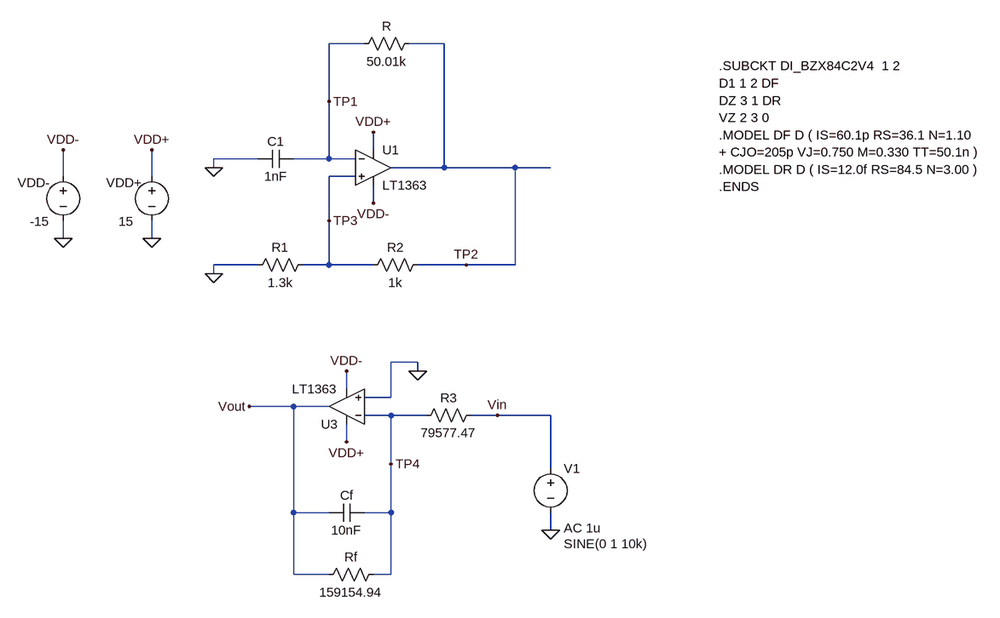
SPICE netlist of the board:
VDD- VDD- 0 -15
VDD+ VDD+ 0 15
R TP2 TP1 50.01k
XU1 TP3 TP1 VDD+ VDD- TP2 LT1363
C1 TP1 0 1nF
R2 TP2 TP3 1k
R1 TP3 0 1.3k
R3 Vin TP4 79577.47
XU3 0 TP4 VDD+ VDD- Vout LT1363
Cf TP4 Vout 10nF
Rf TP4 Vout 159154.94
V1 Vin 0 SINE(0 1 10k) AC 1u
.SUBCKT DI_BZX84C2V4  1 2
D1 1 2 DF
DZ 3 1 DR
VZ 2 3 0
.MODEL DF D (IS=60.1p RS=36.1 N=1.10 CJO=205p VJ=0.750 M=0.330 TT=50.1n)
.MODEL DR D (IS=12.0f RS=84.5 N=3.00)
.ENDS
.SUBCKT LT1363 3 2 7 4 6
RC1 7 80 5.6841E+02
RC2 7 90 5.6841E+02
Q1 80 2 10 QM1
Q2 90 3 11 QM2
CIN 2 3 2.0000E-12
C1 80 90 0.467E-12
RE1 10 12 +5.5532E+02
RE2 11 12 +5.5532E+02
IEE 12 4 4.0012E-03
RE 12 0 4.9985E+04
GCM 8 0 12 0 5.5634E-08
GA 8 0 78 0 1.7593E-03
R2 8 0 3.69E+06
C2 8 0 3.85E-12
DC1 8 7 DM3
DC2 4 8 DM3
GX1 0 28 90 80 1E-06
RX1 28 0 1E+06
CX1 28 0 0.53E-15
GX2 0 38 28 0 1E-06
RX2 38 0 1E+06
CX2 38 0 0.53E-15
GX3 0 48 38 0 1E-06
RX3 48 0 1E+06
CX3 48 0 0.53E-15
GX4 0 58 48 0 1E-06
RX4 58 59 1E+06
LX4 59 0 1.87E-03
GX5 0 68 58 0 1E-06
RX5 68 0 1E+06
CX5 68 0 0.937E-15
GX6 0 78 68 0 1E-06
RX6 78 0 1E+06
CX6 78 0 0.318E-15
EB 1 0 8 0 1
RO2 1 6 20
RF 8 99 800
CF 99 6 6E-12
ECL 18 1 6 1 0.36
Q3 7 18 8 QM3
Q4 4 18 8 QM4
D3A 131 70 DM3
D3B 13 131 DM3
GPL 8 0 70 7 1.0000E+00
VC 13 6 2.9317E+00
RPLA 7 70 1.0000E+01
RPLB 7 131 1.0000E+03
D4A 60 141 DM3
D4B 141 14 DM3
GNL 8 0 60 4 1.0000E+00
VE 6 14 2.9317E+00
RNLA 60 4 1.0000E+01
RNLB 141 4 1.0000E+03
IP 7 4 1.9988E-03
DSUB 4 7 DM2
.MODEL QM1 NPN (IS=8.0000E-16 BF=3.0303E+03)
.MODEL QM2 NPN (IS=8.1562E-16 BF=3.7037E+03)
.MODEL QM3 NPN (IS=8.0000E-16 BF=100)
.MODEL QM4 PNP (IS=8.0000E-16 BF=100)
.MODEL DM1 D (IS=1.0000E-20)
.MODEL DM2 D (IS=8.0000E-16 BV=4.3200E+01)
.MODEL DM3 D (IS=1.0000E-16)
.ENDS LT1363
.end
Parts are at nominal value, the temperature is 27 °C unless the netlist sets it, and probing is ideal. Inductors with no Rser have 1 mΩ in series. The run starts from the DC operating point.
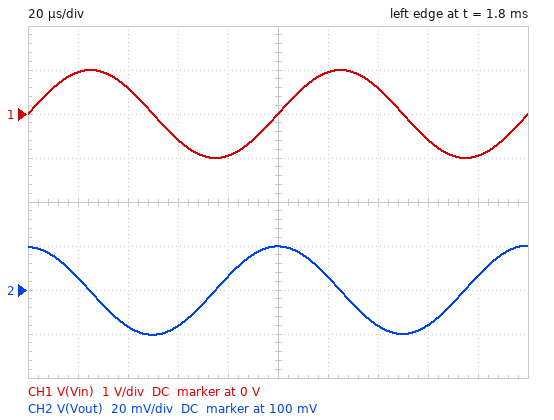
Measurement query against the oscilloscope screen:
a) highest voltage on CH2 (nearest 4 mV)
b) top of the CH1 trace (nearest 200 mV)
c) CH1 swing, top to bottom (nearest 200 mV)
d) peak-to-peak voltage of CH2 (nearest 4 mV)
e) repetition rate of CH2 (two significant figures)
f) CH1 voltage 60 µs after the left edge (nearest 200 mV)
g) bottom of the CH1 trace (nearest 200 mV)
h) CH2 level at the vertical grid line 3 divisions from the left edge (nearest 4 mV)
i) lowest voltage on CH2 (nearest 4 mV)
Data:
120 mV
1.0 V
2.0 V
40 mV
10 kHz
-600 mV
-1.0 V
84 mV
80 mV
